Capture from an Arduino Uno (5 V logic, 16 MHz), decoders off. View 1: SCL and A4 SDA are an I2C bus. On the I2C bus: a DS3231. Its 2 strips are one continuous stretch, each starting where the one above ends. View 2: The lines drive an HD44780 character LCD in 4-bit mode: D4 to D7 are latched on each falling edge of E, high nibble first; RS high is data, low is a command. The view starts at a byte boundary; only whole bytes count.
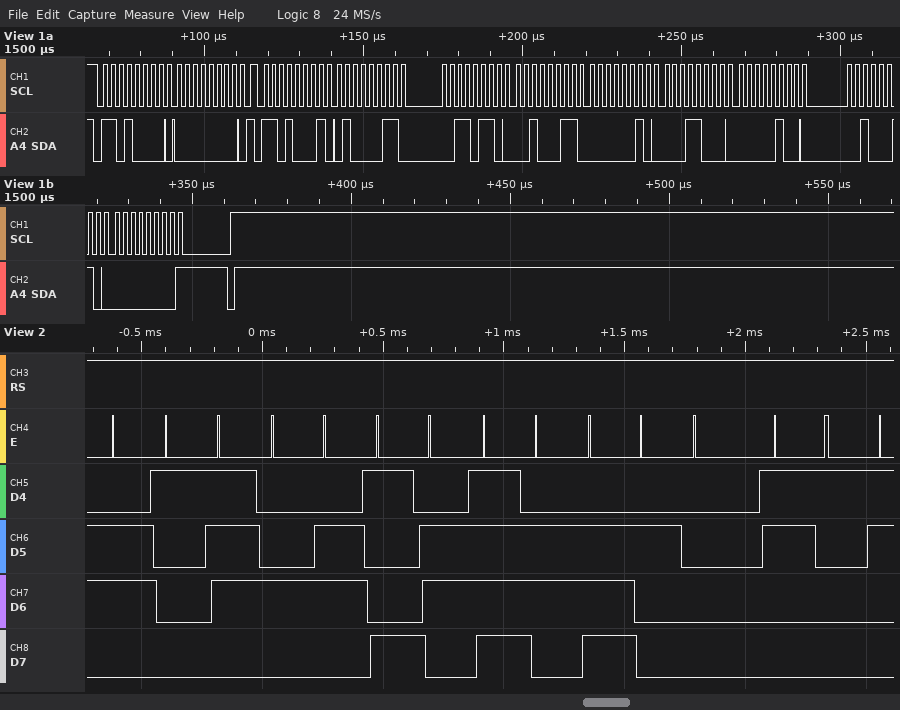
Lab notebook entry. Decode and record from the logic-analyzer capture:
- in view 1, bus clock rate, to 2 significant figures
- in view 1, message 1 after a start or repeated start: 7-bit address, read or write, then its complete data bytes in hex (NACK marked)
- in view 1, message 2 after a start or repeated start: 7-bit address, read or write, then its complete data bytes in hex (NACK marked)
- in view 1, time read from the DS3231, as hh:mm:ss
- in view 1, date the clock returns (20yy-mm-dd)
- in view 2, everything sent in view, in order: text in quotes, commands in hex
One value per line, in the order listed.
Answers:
400 kHz
0x68 write: 00
0x68 read: 43 36 23 02 18 04 22 00 NACK
23:36:43
2022-04-18
"ation 1"
